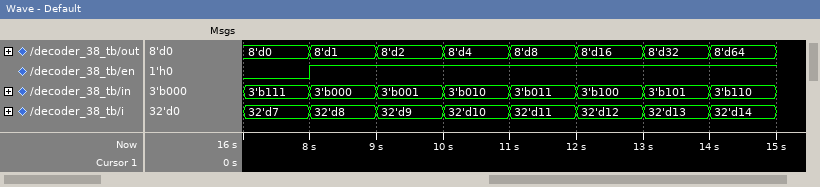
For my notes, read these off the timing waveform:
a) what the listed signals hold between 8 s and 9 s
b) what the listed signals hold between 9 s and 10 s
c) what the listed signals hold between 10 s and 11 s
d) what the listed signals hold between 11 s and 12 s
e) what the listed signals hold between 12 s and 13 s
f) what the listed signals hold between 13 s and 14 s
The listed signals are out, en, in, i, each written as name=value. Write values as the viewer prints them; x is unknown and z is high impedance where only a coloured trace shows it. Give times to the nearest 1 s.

out=8'd1, en=1, in=3'b000, i=32'd8
out=8'd2, en=1, in=3'b001, i=32'd9
out=8'd4, en=1, in=3'b010, i=32'd10
out=8'd8, en=1, in=3'b011, i=32'd11
out=8'd16, en=1, in=3'b100, i=32'd12
out=8'd32, en=1, in=3'b101, i=32'd13
